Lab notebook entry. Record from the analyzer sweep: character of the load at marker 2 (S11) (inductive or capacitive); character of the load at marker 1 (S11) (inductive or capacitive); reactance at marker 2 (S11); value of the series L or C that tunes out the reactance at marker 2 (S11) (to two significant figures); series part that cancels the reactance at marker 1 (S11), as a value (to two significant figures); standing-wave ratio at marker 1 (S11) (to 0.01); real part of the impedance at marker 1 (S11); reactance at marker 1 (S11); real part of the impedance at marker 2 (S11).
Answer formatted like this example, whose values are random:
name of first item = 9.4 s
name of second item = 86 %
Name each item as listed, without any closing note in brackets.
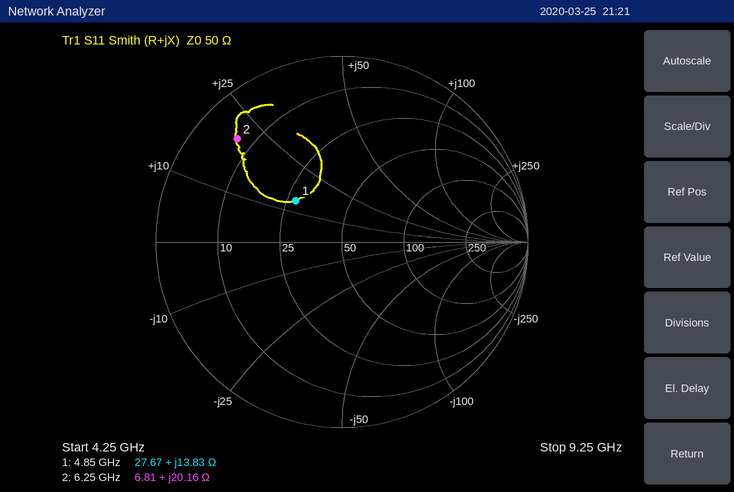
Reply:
character of the load at marker 2 (S11) = inductive
character of the load at marker 1 (S11) = inductive
reactance at marker 2 = +20.16 Ω
value of the series L or C that tunes out the reactance at marker 2 (S11) = 1.3 pF
series part that cancels the reactance at marker 1 (S11), as a value = 2.4 pF
standing-wave ratio at marker 1 (S11) = 2.00
real part of the impedance at marker 1 = 27.67 Ω
reactance at marker 1 = +13.83 Ω
real part of the impedance at marker 2 = 6.81 Ω
